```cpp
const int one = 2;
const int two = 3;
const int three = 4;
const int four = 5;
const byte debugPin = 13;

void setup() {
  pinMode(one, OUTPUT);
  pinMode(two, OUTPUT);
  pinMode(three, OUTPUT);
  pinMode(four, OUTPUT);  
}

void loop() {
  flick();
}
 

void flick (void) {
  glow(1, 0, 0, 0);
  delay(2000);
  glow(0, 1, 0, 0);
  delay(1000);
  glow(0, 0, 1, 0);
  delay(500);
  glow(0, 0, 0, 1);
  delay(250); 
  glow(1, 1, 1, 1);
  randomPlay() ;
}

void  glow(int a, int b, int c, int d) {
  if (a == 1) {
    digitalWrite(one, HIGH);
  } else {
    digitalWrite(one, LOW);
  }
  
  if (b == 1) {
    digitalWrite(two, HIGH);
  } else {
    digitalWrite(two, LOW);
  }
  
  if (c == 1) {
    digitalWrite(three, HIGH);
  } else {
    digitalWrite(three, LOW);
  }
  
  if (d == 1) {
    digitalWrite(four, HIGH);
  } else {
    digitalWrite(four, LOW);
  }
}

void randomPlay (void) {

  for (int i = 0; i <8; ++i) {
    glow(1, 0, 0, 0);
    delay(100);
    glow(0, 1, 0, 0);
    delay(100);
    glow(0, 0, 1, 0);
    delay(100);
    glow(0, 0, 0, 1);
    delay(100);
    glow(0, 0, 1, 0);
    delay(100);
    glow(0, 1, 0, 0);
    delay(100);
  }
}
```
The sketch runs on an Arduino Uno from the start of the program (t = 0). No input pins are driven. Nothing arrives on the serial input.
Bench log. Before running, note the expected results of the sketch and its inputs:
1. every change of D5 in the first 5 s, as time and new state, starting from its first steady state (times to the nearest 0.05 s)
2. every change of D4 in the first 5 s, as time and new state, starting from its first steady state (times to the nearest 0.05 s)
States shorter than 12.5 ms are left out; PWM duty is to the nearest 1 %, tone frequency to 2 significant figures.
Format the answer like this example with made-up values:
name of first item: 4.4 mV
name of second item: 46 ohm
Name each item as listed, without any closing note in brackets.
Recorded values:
every change of D5 in the first 5 s, as time and new state, starting from its first steady state: 0 s low; 3.5 s high; 3.75 s low; 4.05 s high; 4.15 s low; 4.65 s high; 4.75 s low
every change of D4 in the first 5 s, as time and new state, starting from its first steady state: 0 s low; 3 s high; 3.5 s low; 3.95 s high; 4.05 s low; 4.15 s high; 4.25 s low; 4.55 s high; 4.65 s low; 4.75 s high; 4.85 s low
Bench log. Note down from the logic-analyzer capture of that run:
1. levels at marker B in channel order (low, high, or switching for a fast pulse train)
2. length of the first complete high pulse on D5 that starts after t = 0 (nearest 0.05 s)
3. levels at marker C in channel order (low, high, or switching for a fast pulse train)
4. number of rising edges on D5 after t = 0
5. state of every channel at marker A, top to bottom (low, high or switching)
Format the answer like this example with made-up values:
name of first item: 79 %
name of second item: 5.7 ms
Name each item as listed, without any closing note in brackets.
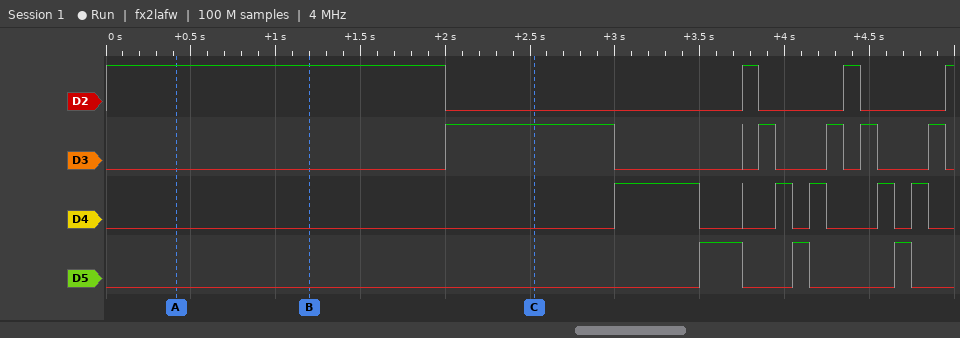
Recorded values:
levels at marker B in channel order: D2 high, D3 low, D4 low, D5 low
length of the first complete high pulse on D5 that starts after t = 0: 0.25 s
levels at marker C in channel order: D2 low, D3 high, D4 low, D5 low
number of rising edges on D5 after t = 0: 3
state of every channel at marker A, top to bottom: D2 high, D3 low, D4 low, D5 low
